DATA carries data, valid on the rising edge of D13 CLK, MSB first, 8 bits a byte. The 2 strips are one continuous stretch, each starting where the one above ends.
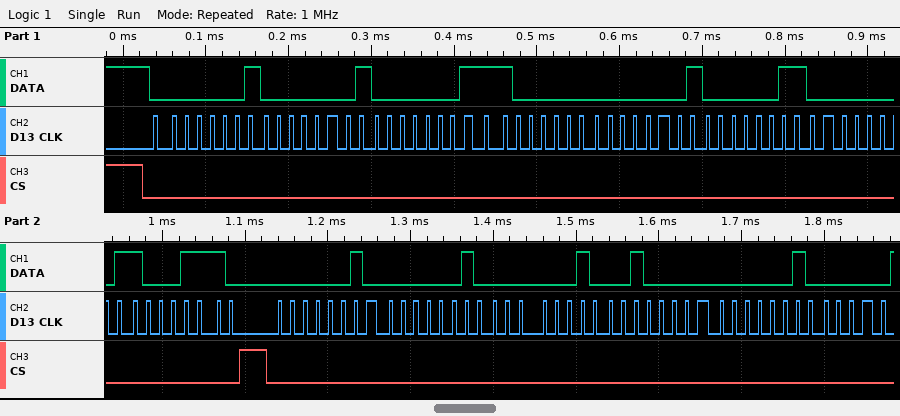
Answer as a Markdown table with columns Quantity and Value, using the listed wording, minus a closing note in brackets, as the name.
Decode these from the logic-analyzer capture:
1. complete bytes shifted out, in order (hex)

| Quantity | Value |
|---|---|
| complete bytes shifted out, in order | 0x01 0x01 0x01 0xC0 0x01 0x03 0x01 0x8E 0x02 0x02 0x02 0x20 0x02 |
